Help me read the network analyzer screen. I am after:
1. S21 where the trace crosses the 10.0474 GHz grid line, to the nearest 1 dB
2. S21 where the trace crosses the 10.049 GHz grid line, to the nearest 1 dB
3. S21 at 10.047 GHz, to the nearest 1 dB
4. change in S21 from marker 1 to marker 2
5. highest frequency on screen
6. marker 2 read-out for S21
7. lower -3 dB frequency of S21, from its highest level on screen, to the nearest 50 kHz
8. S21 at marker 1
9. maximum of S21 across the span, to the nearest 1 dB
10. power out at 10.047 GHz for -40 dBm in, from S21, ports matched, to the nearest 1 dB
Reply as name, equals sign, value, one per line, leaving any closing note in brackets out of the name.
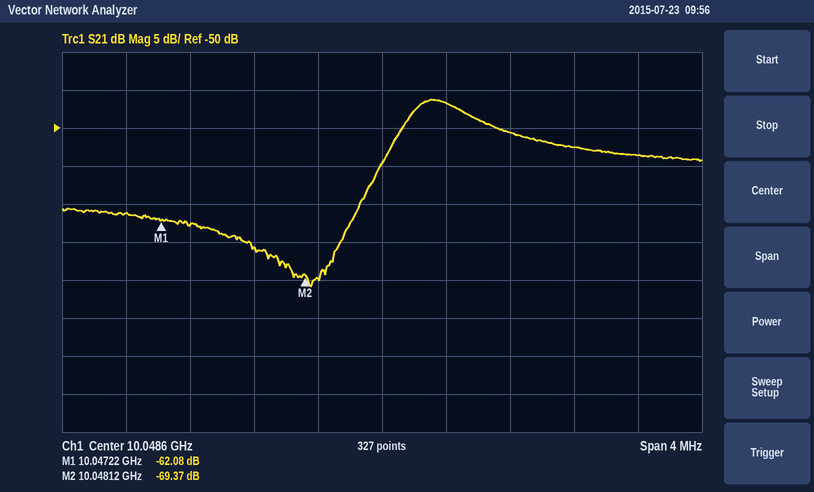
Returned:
S21 where the trace crosses the 10.0474 GHz grid line, to the nearest 1 dB = -63 dB
S21 where the trace crosses the 10.049 GHz grid line, to the nearest 1 dB = -47 dB
S21 at 10.047 GHz, to the nearest 1 dB = -61 dB
change in S21 from marker 1 to marker 2 = -7.29 dB
highest frequency on screen = 10.0506 GHz
marker 2 read-out for S21 = -69.37 dB
lower -3 dB frequency of S21, from its highest level on screen, to the nearest 50 kHz = 10.04875 GHz
S21 at marker 1 = -62.08 dB
maximum of S21 across the span, to the nearest 1 dB = -46 dB
power out at 10.047 GHz for -40 dBm in, from S21, ports matched, to the nearest 1 dB = -101 dBm
